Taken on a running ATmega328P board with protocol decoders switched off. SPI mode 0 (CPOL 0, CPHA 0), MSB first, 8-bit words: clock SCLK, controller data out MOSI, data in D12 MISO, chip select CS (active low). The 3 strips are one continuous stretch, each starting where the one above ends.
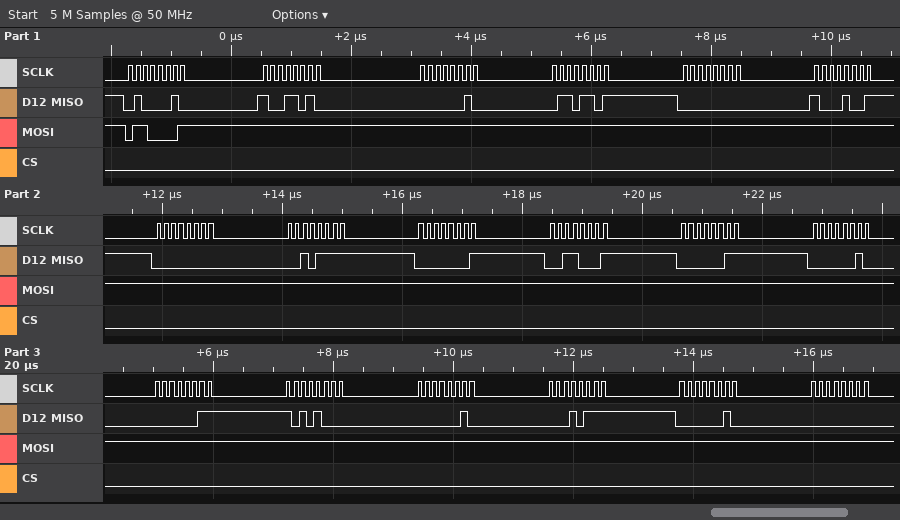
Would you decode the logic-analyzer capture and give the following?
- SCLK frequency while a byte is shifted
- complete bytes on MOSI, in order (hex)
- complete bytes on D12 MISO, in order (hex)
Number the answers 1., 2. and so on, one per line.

1. 8 MHz
2. 61 FF FF FF FF FF FF FF FF FF FF FF FF FF FF FF FF FF
3. 42 9A 02 6D 00 89 00 2F 01 31 03 02 03 A8 02 17 02 00
